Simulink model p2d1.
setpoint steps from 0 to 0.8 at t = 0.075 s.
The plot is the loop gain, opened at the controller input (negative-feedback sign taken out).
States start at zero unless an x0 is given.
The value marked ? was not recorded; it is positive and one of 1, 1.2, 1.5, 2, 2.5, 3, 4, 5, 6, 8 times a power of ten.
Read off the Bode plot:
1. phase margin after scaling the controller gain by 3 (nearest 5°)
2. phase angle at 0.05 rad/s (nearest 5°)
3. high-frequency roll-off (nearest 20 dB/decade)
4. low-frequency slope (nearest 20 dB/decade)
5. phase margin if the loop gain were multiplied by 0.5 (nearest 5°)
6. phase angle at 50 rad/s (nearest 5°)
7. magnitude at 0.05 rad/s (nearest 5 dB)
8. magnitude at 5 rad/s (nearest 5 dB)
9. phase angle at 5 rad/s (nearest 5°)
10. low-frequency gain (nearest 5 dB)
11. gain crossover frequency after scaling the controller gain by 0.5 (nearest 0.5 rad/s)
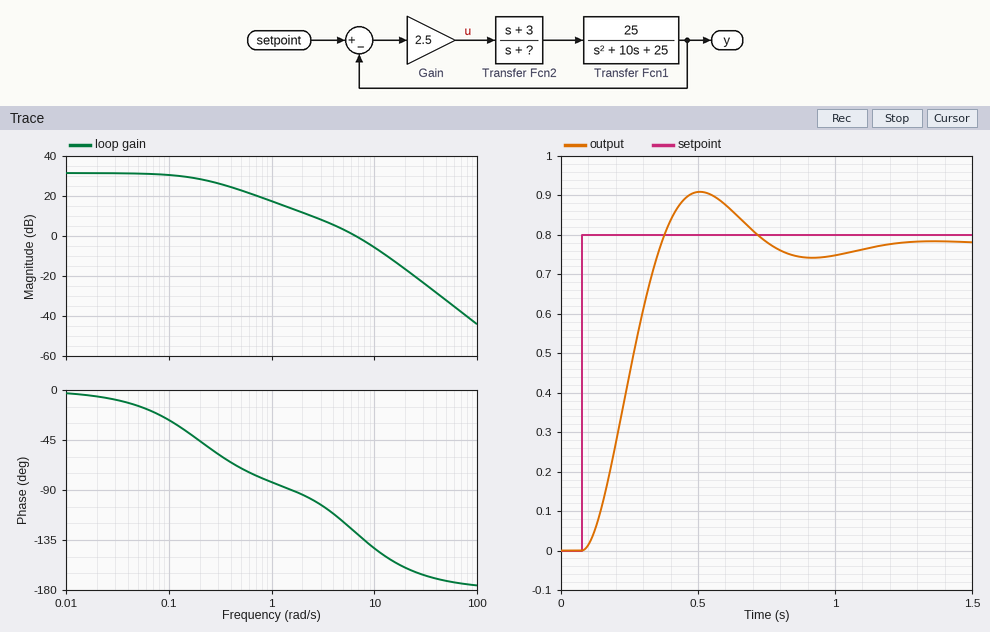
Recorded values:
30°
-15°
-40 dB/decade
0 dB/decade
70°
-170°
30 dB
5 dB
-120°
30 dB
4.0 rad/s
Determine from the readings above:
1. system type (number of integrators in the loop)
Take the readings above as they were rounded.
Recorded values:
0
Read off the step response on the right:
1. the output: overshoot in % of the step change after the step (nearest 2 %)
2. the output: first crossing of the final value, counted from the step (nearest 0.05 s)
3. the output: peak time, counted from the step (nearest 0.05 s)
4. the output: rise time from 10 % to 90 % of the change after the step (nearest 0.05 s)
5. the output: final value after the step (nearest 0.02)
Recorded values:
16 %
0.30 s
0.45 s
0.20 s
0.78
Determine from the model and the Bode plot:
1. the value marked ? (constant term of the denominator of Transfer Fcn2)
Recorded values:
0.2
